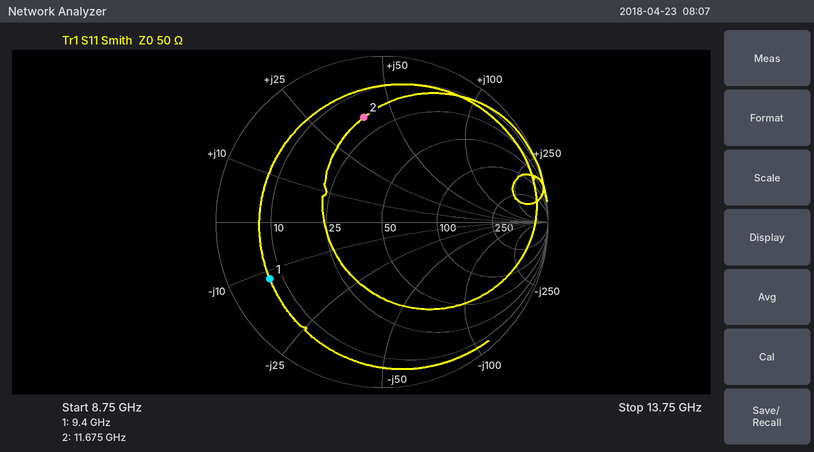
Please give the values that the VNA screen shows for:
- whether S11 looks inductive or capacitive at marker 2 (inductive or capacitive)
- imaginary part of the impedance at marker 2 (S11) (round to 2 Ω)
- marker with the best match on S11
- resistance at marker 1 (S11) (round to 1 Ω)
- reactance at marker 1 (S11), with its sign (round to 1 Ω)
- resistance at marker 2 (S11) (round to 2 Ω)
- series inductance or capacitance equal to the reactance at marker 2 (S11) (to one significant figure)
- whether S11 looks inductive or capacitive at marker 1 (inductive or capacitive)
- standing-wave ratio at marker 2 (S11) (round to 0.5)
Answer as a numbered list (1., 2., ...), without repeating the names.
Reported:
1. inductive
2. +38 Ω
3. marker 2
4. 7 Ω
5. -12 Ω
6. 18 Ω
7. 500 pH
8. capacitive
9. 4.5
